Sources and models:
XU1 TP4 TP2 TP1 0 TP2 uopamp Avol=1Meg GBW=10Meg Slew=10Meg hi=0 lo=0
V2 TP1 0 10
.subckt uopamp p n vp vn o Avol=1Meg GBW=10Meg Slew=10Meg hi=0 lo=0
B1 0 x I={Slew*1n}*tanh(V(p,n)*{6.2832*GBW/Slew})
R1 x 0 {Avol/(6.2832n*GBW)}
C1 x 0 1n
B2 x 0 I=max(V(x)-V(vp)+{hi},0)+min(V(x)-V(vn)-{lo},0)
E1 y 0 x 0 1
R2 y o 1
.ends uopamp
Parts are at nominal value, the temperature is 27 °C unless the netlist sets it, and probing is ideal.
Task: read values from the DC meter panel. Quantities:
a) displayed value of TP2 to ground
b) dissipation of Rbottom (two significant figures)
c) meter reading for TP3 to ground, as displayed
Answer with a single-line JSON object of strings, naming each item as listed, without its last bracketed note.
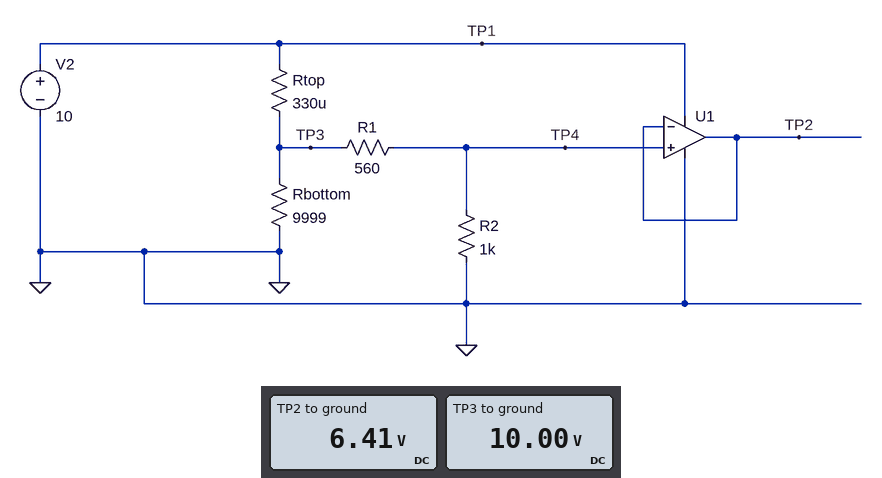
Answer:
{"displayed value of TP2 to ground": "6.41 V", "dissipation of Rbottom": "10 mW", "meter reading for TP3 to ground, as displayed": "10.00 V"}
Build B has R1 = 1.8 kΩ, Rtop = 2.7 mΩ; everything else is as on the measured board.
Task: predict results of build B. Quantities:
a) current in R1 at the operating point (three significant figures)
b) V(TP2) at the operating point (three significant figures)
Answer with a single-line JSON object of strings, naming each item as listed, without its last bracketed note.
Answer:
{"current in R1 at the operating point": "3.57 mA", "V(TP2) at the operating point": "3.57 V"}
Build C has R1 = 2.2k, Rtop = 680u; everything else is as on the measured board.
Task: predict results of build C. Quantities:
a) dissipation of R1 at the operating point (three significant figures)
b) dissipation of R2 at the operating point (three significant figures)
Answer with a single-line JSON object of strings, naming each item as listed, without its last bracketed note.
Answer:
{"dissipation of R1 at the operating point": "21.5 mW", "dissipation of R2 at the operating point": "9.77 mW"}
